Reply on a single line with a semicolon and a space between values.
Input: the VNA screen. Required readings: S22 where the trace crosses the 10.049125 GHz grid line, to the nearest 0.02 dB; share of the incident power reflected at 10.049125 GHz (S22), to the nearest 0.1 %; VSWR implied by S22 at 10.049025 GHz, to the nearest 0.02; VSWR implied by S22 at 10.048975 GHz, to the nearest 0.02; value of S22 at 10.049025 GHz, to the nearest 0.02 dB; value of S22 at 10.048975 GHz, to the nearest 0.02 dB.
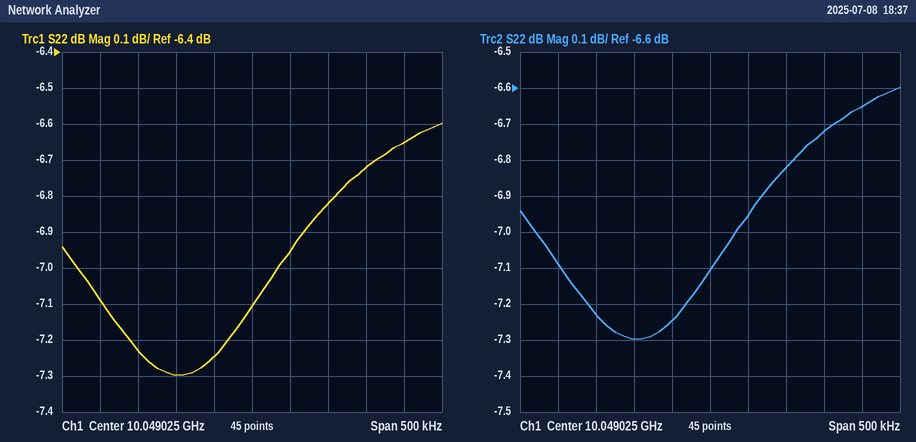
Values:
-6.82 dB; 20.8 %; 2.58; 2.54; -7.10 dB; -7.24 dB
